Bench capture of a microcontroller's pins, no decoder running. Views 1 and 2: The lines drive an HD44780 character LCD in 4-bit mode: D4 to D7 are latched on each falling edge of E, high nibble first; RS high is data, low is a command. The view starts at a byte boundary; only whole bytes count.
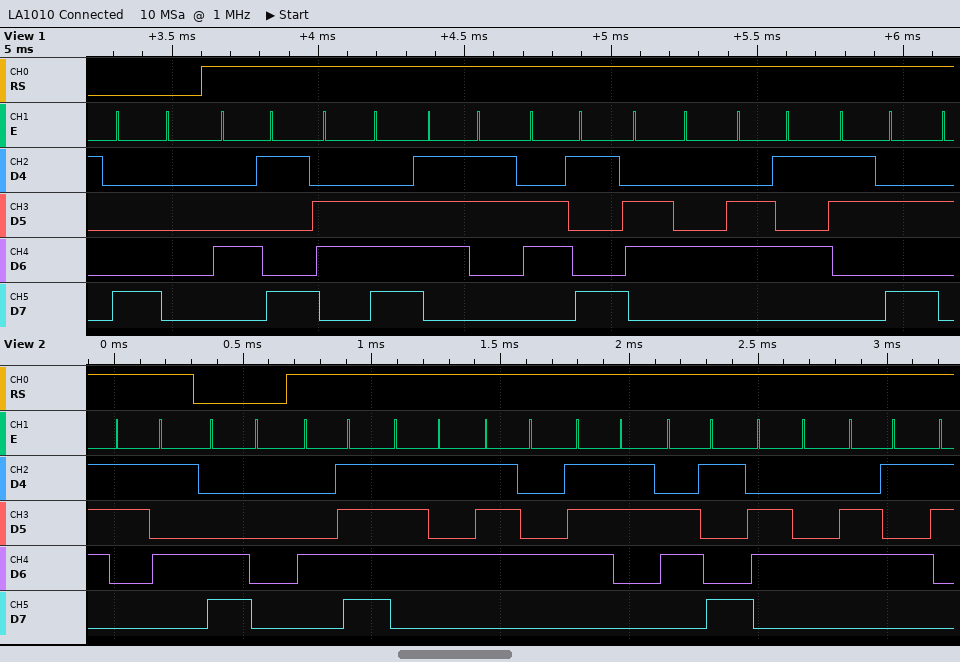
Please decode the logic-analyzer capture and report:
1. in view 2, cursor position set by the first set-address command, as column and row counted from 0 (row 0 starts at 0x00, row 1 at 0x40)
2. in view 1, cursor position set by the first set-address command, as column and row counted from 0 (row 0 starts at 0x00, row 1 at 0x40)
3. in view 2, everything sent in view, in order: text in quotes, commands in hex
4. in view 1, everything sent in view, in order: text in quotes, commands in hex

column 0, row 1
column 0, row 0
"5" 0xC0 "Outside"
0x80 "Inside:"
